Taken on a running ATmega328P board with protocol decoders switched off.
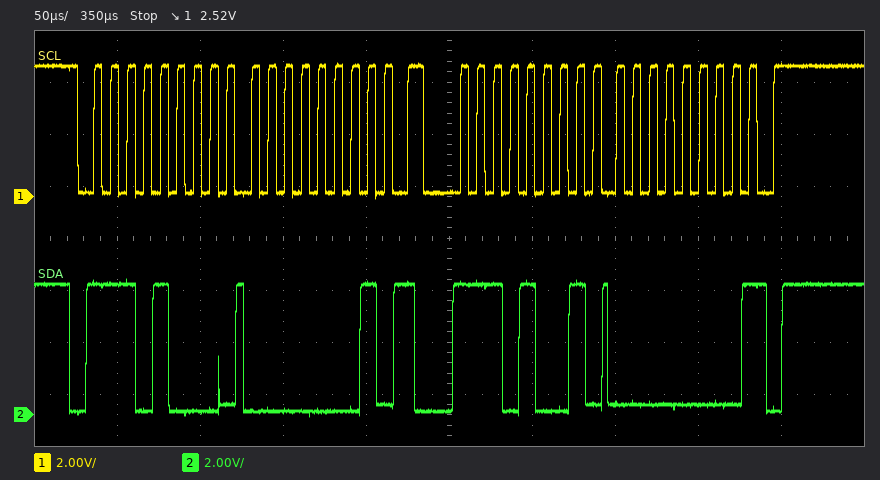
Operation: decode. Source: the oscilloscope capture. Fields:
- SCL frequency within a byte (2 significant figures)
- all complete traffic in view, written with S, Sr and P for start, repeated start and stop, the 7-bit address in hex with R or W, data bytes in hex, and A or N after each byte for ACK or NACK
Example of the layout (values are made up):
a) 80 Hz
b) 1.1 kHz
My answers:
a) 100 kHz
b) S 74W A 01 A Sr 74R A 00 N P
